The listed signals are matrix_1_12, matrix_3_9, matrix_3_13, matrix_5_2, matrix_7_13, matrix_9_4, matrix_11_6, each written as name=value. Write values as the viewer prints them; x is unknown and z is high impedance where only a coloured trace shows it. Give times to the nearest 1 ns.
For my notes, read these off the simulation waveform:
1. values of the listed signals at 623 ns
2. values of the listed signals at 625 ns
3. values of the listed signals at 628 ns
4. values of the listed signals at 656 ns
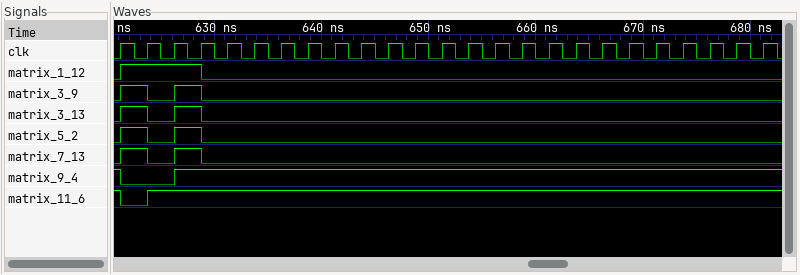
matrix_1_12=1, matrix_3_9=1, matrix_3_13=1, matrix_5_2=1, matrix_7_13=1, matrix_9_4=0, matrix_11_6=0
matrix_1_12=1, matrix_3_9=0, matrix_3_13=0, matrix_5_2=0, matrix_7_13=0, matrix_9_4=0, matrix_11_6=1
matrix_1_12=1, matrix_3_9=1, matrix_3_13=1, matrix_5_2=1, matrix_7_13=1, matrix_9_4=1, matrix_11_6=1
matrix_1_12=0, matrix_3_9=0, matrix_3_13=0, matrix_5_2=0, matrix_7_13=0, matrix_9_4=1, matrix_11_6=1
